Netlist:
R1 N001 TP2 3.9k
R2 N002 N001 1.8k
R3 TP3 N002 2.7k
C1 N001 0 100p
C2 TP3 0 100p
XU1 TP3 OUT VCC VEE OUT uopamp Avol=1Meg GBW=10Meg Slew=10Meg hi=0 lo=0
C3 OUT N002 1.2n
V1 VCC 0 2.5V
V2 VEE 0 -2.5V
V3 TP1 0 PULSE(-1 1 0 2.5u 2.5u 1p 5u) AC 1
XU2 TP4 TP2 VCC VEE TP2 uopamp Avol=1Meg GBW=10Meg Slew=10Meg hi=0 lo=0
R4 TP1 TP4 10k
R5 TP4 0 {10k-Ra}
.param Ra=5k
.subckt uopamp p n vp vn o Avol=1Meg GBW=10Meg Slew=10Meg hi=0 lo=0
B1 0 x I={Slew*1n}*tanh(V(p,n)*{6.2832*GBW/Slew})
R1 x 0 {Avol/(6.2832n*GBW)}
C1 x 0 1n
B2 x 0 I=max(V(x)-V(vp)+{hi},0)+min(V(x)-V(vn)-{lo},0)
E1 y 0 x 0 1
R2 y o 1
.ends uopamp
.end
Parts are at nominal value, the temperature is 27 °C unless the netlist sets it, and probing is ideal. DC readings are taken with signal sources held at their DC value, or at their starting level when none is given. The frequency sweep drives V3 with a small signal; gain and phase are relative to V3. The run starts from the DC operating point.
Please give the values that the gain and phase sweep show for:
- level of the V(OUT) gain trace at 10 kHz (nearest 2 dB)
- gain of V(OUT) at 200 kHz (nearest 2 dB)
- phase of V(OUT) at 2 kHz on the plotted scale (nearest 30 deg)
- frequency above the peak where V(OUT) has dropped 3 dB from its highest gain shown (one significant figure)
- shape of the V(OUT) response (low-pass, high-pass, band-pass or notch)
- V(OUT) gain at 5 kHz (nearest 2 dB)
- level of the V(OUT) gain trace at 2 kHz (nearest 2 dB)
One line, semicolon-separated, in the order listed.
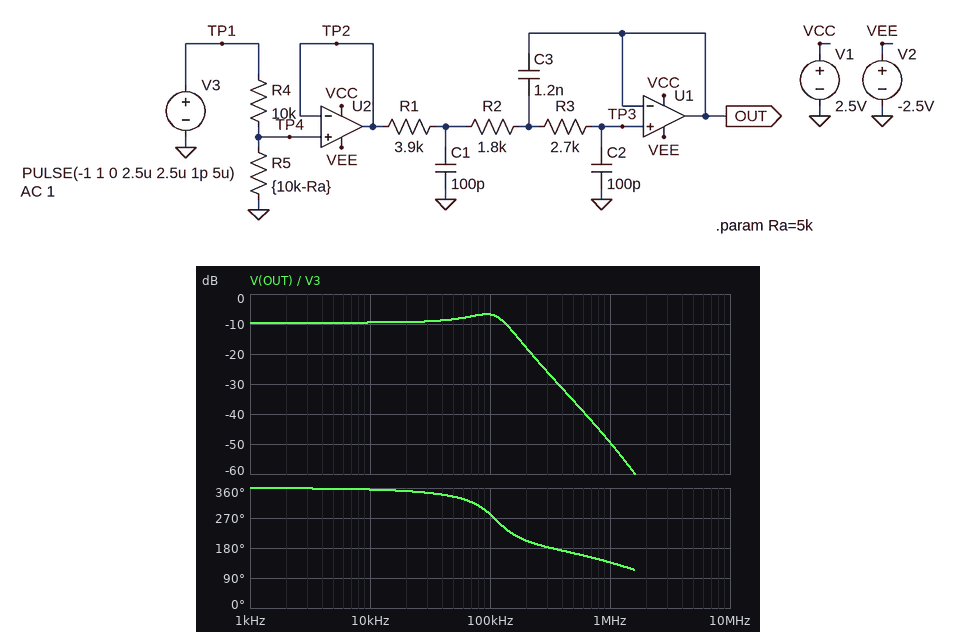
-10 dB; -18 dB; 360 deg; 100 kHz; low-pass; -10 dB; -10 dB
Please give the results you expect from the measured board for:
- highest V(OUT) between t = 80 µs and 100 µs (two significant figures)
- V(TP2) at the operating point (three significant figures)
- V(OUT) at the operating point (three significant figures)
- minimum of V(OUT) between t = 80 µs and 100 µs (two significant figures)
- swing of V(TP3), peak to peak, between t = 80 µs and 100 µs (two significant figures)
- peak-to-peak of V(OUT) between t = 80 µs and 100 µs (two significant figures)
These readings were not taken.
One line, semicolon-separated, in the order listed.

100 mV; -333 mV; -333 mV; -100 mV; 210 mV; 210 mV
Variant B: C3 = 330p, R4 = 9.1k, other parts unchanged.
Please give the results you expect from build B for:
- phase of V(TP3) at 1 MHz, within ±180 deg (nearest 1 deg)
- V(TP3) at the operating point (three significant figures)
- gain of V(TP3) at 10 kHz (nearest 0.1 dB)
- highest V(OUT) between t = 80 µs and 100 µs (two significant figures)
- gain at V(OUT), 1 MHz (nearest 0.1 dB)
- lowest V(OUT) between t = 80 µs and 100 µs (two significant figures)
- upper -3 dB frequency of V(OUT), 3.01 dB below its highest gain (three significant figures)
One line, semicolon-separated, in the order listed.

157 deg; -355 mV; -9.0 dB; 200 mV; -38.2 dB; -200 mV; 199 kHz
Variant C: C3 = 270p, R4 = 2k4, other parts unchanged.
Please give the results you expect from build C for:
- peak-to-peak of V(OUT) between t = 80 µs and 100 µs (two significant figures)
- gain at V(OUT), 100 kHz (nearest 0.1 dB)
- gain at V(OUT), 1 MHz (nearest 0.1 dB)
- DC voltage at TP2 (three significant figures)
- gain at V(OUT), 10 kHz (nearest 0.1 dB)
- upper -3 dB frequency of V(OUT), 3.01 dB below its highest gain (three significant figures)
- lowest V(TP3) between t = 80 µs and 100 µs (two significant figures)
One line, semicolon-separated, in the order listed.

760 mV; -4.0 dB; -31.1 dB; -676 mV; -3.4 dB; 196 kHz; -380 mV
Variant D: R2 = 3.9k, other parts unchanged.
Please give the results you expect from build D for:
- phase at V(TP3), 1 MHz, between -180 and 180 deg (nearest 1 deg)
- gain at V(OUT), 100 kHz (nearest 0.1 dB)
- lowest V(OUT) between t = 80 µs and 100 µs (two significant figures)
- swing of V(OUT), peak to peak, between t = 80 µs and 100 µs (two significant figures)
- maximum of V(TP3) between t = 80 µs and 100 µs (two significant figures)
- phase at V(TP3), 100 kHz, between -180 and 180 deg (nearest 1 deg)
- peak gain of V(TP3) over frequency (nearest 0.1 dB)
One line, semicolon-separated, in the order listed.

128 deg; -7.5 dB; -73 mV; 150 mV; 73 mV; -102 deg; -6.5 dB
